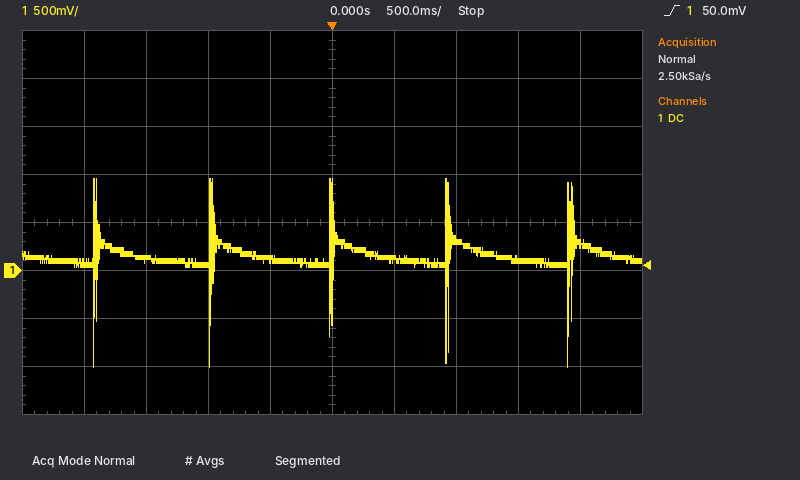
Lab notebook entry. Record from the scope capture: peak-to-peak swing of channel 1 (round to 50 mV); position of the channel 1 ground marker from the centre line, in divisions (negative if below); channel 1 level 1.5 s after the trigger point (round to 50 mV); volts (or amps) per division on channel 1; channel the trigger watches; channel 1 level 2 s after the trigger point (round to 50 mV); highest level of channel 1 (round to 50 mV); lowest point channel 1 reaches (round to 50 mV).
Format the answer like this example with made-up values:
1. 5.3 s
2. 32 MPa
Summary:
1. 1.95 V
2. -1.0 div
3. 100 mV
4. 500 mV
5. channel 1
6. 300 mV
7. 950 mV
8. -1.00 V
